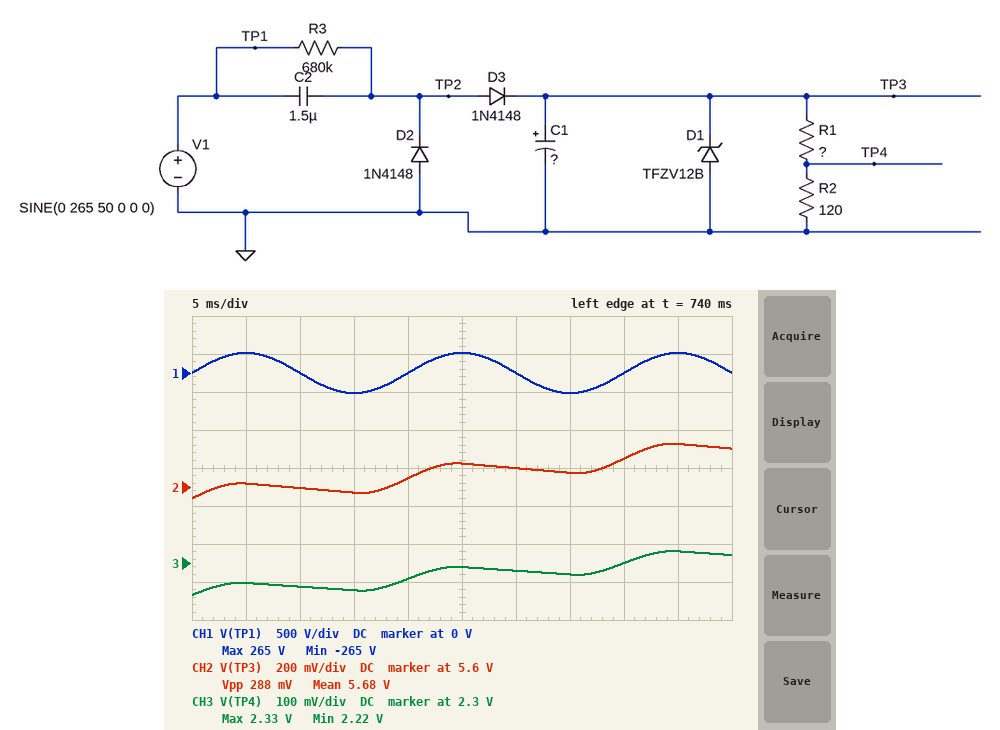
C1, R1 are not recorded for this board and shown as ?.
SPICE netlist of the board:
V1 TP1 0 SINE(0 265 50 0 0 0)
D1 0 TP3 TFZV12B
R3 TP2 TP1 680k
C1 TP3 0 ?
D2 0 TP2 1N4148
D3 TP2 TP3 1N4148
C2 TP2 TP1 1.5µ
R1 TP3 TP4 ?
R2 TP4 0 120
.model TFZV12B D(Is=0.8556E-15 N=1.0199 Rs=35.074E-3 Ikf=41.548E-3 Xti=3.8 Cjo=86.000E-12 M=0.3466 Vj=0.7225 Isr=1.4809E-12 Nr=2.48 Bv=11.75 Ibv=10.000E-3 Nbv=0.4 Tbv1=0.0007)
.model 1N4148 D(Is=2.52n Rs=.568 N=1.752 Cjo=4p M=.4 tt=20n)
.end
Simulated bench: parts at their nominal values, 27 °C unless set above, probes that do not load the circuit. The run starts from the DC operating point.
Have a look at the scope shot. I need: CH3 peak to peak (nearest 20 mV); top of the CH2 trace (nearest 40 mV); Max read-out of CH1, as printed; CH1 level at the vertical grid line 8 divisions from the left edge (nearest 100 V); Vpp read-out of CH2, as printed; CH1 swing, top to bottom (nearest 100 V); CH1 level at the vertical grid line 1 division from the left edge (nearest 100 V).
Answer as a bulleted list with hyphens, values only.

- 120 mV
- 5.84 V
- 265 V
- 0 V
- 288 mV
- 500 V
- 300 V
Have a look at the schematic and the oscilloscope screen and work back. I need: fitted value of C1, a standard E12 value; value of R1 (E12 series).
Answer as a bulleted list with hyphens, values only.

- 3.9 mF
- 180 Ω
